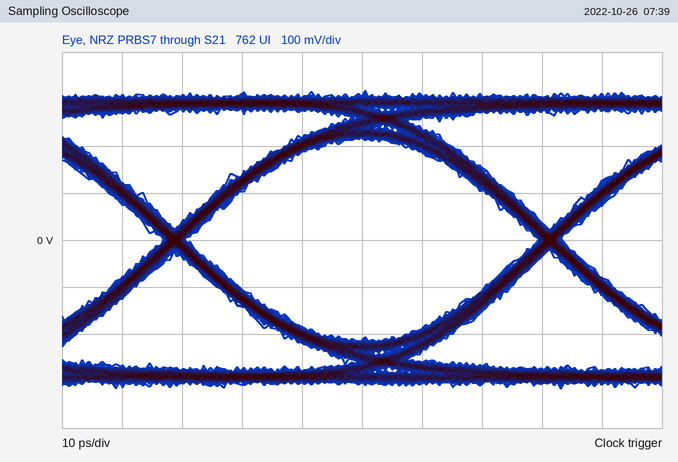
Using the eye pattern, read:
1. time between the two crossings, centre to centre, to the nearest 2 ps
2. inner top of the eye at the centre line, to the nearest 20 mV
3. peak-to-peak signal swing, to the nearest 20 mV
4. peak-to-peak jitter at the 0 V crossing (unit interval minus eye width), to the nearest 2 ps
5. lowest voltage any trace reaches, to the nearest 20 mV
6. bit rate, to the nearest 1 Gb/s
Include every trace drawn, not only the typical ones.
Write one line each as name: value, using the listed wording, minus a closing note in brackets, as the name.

time between the two crossings, centre to centre, to the nearest 2 ps: 62 ps
inner top of the eye at the centre line, to the nearest 20 mV: 220 mV
peak-to-peak signal swing, to the nearest 20 mV: 640 mV
peak-to-peak jitter at the 0 V crossing (unit interval minus eye width), to the nearest 2 ps: 4 ps
lowest voltage any trace reaches, to the nearest 20 mV: -320 mV
bit rate, to the nearest 1 Gb/s: 16 Gb/s
